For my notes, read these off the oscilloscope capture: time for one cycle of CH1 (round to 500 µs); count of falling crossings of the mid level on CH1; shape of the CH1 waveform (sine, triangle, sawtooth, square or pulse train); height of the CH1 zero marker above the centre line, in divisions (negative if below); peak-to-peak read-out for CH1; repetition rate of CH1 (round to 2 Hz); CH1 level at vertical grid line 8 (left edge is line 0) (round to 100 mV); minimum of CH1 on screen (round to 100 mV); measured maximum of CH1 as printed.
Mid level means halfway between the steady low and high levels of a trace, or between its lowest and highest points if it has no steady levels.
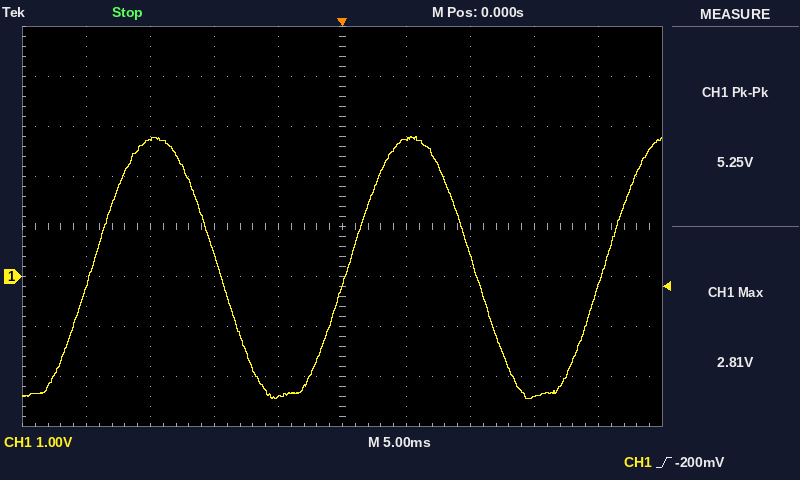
20.0 ms
2
sine
-1.0 div
5.25 V
50 Hz
-2.4 V
-2.4 V
2.81 V
